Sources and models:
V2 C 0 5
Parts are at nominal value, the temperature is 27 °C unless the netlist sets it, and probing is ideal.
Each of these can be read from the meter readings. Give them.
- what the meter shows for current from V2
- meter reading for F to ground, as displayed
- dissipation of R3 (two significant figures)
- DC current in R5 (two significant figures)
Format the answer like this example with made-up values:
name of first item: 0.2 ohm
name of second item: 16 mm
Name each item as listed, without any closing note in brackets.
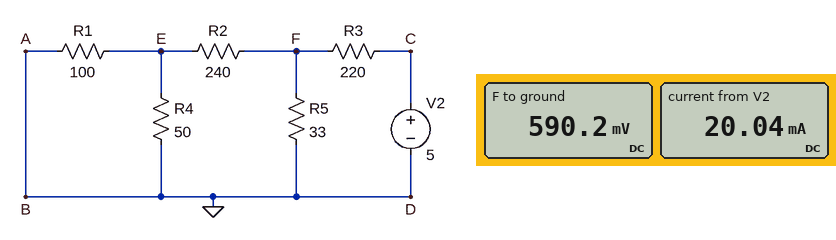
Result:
what the meter shows for current from V2: 20.04 mA
meter reading for F to ground, as displayed: 590.2 mV
dissipation of R3: 88 mW
DC current in R5: 18 mA
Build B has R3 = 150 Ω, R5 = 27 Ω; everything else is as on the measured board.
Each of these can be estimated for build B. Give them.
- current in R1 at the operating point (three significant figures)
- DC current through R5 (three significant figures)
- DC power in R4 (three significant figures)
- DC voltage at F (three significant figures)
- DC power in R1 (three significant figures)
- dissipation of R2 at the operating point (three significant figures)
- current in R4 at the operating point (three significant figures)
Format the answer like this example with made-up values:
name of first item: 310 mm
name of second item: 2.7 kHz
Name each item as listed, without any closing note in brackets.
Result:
current in R1 at the operating point: 858 µA
DC current through R5: 26.1 mA
DC power in R4: 147 µW
DC voltage at F: 704 mV
DC power in R1: 73.7 µW
dissipation of R2 at the operating point: 1.59 mW
current in R4 at the operating point: 1.72 mA
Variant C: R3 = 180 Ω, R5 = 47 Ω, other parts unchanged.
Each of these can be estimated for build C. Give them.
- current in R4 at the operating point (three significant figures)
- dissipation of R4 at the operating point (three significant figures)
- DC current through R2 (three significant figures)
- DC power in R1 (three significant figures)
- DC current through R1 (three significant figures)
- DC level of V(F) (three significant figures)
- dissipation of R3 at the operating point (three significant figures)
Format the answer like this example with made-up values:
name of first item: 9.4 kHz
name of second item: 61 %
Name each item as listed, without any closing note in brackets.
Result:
current in R4 at the operating point: 2.22 mA
dissipation of R4 at the operating point: 247 µW
DC current through R2: 3.33 mA
DC power in R1: 123 µW
DC current through R1: 1.11 mA
DC level of V(F): 911 mV
dissipation of R3 at the operating point: 92.9 mW
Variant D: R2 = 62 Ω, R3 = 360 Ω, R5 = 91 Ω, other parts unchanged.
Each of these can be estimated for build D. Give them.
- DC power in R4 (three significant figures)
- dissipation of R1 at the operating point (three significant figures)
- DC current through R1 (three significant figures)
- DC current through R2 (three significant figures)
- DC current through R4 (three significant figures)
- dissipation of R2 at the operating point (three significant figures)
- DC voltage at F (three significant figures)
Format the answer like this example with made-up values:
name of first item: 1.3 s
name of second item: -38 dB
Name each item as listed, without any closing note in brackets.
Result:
DC power in R4: 802 µW
dissipation of R1 at the operating point: 401 µW
DC current through R1: 2.00 mA
DC current through R2: 6.01 mA
DC current through R4: 4.00 mA
dissipation of R2 at the operating point: 2.24 mW
DC voltage at F: 573 mV
